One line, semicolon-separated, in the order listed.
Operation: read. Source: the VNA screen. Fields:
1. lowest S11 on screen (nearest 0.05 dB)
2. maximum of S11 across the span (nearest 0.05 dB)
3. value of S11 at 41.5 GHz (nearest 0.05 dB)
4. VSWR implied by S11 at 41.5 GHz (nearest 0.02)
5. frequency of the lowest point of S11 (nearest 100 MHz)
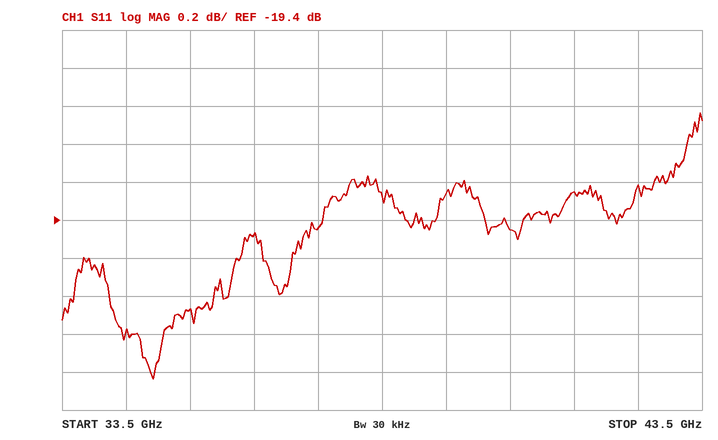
-20.25 dB; -18.85 dB; -19.25 dB; 1.24; 34.9 GHz
